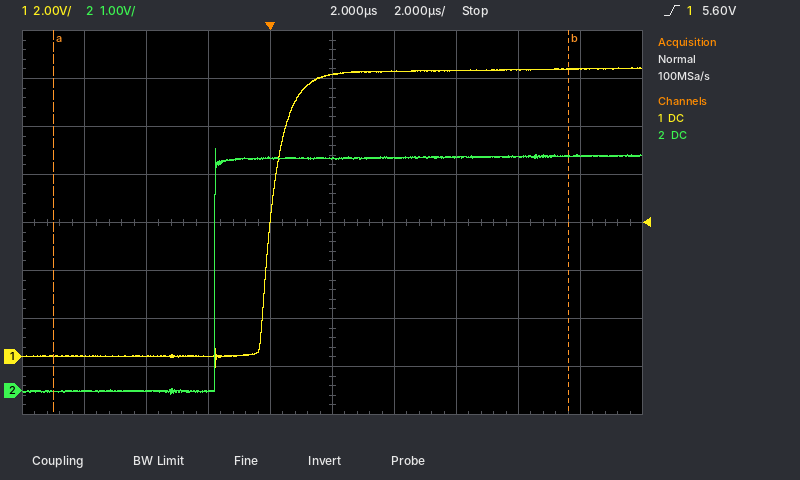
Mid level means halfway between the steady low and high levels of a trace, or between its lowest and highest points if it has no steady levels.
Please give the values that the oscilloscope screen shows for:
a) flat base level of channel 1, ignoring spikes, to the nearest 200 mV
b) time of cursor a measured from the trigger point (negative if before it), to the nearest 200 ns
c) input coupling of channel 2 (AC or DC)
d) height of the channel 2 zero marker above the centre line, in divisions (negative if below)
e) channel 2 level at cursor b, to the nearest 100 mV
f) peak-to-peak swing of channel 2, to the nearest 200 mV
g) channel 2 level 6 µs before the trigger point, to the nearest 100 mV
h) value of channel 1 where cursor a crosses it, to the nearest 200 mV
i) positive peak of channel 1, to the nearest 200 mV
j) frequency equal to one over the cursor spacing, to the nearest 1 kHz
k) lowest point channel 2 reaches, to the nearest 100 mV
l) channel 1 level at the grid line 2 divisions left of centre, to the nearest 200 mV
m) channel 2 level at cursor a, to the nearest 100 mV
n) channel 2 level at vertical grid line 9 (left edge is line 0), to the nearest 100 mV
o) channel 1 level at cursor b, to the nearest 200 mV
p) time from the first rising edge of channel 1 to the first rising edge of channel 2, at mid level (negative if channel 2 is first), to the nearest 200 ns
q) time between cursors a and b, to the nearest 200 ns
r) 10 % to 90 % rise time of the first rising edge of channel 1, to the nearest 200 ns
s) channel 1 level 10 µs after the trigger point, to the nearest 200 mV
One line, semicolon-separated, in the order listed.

0.0 V; -7.0 µs; DC; -3.5 div; 4.9 V; 5.2 V; 0.0 V; 0.0 V; 12.0 V; 60 kHz; -100 mV; 0.0 V; 0.0 V; 4.9 V; 12.0 V; -1.8 µs; 16.6 µs; 1.2 µs; 12.0 V
